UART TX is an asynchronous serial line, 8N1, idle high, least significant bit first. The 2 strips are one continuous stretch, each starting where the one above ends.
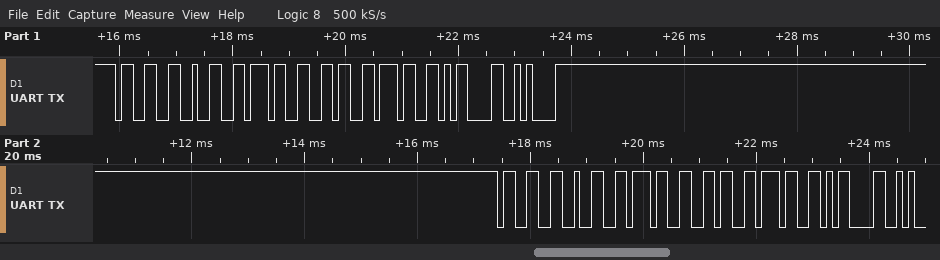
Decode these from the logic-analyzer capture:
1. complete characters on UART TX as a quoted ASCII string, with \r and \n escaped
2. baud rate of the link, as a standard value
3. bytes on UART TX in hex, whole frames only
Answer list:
"32767\r\n32767\r"
9600 baud
0x33 0x32 0x37 0x36 0x37 0x0D 0x0A 0x33 0x32 0x37 0x36 0x37 0x0D
